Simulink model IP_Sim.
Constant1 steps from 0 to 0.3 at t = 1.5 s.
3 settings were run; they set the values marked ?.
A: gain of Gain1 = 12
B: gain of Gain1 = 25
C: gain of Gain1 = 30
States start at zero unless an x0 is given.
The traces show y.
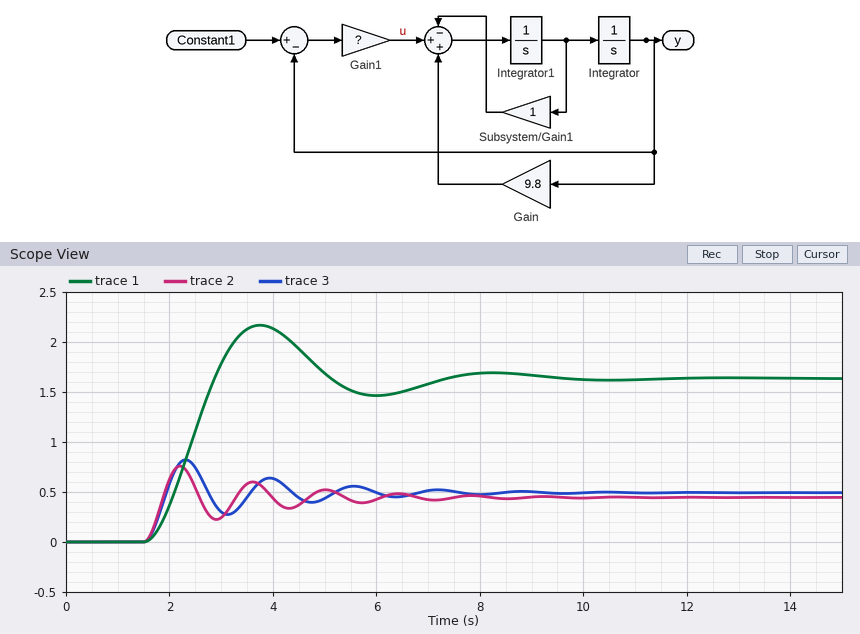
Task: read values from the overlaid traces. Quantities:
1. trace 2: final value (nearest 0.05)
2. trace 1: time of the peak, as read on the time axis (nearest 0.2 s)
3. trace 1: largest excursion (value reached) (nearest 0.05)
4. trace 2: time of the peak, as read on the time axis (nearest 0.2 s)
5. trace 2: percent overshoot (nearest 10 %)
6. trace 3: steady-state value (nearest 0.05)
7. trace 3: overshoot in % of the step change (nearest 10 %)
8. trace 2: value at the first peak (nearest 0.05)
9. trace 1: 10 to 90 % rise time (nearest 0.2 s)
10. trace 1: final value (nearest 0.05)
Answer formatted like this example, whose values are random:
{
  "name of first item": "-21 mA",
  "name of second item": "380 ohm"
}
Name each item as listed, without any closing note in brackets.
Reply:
{
  "trace 2: final value": "0.45",
  "trace 1: time of the peak, as read on the time axis": "3.8 s",
  "trace 1: largest excursion (value reached)": "2.15",
  "trace 2: time of the peak, as read on the time axis": "2.2 s",
  "trace 2: percent overshoot": "70 %",
  "trace 3: steady-state value": "0.50",
  "trace 3: overshoot in % of the step change": "70 %",
  "trace 2: value at the first peak": "0.75",
  "trace 1: 10 to 90 % rise time": "1.0 s",
  "trace 1: final value": "1.65"
}
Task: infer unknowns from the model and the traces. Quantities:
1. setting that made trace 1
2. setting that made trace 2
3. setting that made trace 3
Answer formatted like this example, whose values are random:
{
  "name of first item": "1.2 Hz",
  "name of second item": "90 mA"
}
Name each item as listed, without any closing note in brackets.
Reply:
{
  "setting that made trace 1": "A",
  "setting that made trace 2": "C",
  "setting that made trace 3": "B"
}
